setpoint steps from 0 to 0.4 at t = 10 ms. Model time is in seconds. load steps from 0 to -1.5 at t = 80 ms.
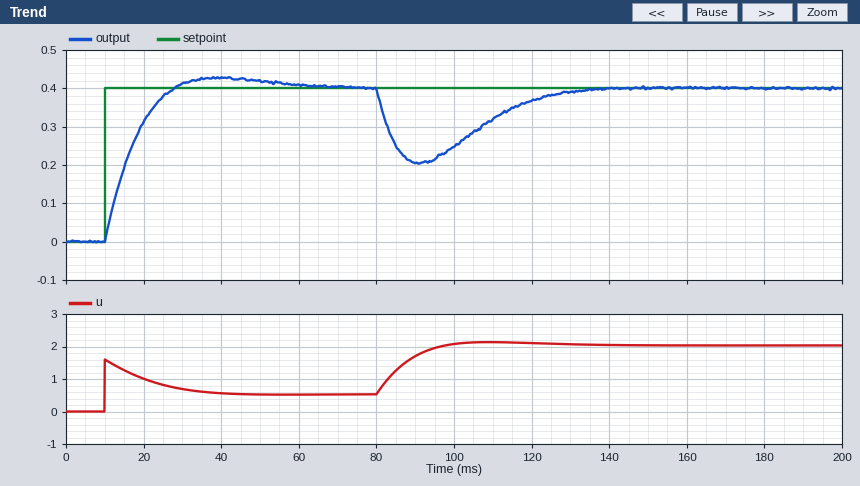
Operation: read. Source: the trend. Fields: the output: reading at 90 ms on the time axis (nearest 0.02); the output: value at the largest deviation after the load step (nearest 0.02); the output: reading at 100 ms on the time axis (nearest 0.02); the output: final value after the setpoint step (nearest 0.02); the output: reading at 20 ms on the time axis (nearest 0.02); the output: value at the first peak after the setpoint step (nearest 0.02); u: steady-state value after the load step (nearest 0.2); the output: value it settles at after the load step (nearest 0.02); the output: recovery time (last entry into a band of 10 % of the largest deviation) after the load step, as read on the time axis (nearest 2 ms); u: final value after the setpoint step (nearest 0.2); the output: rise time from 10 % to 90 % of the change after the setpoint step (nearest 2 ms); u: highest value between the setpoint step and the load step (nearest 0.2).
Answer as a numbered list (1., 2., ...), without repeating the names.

1. 0.20
2. 0.20
3. 0.24
4. 0.40
5. 0.32
6. 0.42
7. 2.0
8. 0.40
9. 124 ms
10. 0.6
11. 12 ms
12. 1.6
